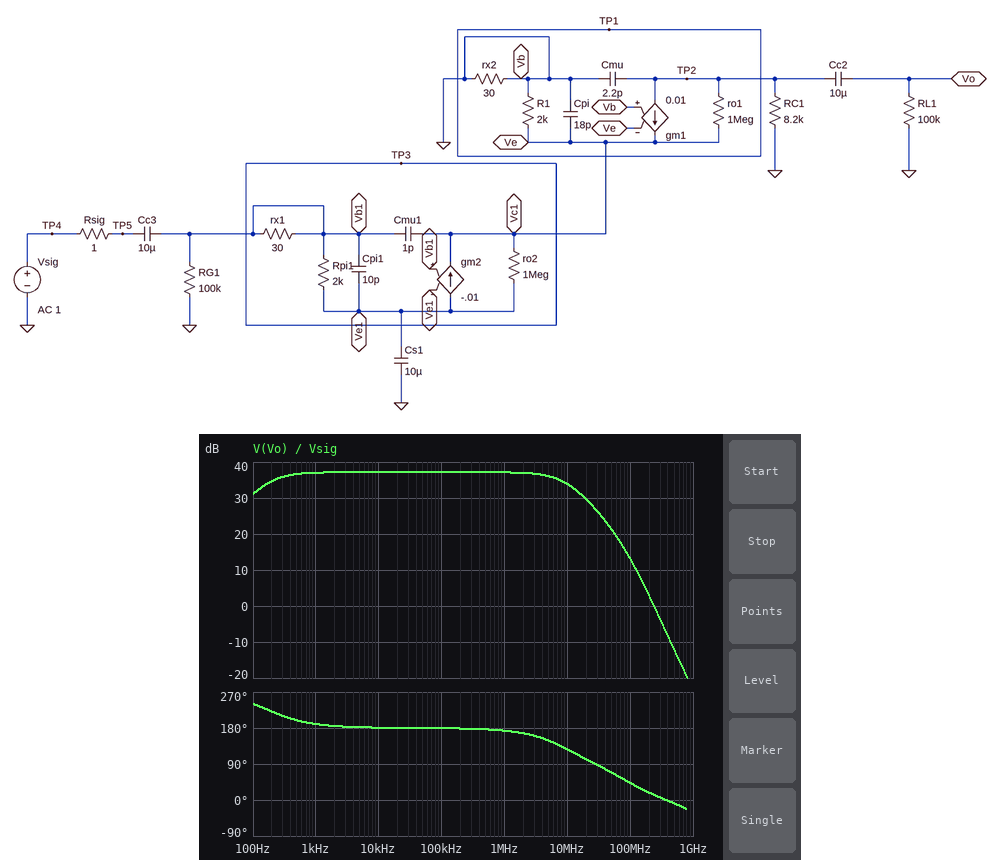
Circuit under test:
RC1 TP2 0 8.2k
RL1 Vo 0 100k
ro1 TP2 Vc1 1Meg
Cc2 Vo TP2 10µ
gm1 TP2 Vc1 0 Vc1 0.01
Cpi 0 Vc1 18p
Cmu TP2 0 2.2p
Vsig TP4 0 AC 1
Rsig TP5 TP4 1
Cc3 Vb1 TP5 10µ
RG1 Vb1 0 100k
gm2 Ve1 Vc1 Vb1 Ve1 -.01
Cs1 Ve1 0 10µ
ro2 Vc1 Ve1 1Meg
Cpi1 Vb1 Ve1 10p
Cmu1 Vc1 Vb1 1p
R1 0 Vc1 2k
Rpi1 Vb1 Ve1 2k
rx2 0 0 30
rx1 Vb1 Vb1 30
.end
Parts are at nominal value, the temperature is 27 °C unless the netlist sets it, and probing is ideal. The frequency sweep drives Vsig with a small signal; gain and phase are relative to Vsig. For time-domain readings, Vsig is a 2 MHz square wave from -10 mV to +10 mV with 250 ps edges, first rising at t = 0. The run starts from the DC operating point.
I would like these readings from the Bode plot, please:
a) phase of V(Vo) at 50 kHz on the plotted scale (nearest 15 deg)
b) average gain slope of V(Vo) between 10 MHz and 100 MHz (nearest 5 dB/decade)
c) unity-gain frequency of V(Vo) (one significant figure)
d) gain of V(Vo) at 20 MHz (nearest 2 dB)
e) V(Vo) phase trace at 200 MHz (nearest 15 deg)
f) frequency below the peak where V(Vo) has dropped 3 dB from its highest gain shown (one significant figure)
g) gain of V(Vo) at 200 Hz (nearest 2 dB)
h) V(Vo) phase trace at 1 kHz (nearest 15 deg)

180 deg
-20 dB/decade
200 MHz
30 dB
15 deg
200 Hz
34 dB
195 deg
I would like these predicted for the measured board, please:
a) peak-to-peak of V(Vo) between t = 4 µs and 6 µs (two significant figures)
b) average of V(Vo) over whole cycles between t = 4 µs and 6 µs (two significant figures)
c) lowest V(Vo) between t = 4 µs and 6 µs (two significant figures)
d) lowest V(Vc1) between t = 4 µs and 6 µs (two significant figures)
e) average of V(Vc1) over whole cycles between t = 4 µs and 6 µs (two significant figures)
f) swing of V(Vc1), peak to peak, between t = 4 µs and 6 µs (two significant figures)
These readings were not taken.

1.4 V
-720 mV
-1.4 V
-19 mV
-9.5 mV
20 mV
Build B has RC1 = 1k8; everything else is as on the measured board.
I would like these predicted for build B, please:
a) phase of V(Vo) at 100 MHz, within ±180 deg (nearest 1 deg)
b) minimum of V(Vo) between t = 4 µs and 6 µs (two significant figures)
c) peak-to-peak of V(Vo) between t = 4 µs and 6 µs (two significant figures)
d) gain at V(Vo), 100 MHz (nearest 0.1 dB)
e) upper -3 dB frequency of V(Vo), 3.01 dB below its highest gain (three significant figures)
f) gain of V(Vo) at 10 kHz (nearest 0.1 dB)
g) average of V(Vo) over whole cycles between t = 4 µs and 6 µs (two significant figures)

60 deg
-340 mV
340 mV
12.5 dB
34.9 MHz
24.5 dB
-170 mV
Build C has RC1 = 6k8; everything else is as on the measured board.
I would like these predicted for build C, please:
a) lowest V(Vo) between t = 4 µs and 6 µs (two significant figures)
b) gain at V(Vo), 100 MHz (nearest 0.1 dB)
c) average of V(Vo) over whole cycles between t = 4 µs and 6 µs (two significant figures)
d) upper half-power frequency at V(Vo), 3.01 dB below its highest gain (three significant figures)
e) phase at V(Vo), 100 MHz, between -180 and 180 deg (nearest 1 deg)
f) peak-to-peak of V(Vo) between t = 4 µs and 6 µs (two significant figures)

-1.2 V
13.1 dB
-600 mV
11.2 MHz
44 deg
1.2 V
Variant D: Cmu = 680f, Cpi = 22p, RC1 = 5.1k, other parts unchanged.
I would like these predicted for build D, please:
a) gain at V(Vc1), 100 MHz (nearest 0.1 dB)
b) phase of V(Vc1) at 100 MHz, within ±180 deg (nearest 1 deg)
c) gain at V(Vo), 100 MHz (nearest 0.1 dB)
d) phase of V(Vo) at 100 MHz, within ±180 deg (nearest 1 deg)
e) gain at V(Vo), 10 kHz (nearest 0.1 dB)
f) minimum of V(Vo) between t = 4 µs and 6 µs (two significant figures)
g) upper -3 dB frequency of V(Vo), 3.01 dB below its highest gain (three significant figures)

-5.0 dB
122 deg
21.4 dB
58 deg
33.3 dB
-920 mV
36.9 MHz
